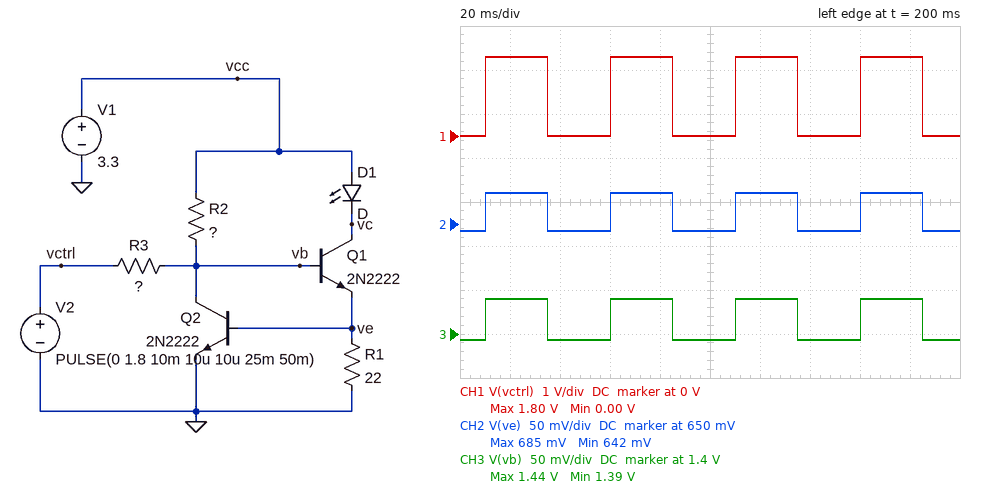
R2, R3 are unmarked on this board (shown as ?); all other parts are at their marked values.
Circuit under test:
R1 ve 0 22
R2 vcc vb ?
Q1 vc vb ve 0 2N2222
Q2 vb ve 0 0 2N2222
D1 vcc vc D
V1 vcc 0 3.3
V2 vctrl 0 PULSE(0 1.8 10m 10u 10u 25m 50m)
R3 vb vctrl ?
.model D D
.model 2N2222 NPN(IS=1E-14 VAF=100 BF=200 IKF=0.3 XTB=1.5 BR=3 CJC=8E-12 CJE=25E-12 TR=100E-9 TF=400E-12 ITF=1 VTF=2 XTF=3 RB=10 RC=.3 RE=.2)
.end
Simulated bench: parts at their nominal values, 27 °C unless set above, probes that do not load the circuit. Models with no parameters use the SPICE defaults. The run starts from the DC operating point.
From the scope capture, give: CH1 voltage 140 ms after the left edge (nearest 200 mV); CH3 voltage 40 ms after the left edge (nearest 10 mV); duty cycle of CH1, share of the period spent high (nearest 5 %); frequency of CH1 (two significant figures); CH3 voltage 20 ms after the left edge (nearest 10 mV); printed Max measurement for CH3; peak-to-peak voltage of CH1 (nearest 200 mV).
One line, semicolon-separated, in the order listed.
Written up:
0 V; 1.39 V; 50 %; 20 Hz; 1.44 V; 1.44 V; 1.8 V
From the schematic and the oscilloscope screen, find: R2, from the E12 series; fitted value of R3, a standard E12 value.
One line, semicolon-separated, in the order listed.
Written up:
680 Ω; 680 Ω
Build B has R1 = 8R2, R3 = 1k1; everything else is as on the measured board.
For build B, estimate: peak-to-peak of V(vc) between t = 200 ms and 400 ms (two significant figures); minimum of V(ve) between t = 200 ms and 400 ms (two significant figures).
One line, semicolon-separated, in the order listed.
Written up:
1.0 mV; 650 mV
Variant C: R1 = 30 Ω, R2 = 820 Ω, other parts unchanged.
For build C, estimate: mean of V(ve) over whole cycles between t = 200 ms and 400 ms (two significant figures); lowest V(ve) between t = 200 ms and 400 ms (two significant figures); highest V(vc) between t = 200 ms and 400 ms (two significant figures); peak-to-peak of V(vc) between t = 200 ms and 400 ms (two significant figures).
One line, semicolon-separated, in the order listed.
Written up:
650 mV; 620 mV; 2.6 V; 2.5 mV
